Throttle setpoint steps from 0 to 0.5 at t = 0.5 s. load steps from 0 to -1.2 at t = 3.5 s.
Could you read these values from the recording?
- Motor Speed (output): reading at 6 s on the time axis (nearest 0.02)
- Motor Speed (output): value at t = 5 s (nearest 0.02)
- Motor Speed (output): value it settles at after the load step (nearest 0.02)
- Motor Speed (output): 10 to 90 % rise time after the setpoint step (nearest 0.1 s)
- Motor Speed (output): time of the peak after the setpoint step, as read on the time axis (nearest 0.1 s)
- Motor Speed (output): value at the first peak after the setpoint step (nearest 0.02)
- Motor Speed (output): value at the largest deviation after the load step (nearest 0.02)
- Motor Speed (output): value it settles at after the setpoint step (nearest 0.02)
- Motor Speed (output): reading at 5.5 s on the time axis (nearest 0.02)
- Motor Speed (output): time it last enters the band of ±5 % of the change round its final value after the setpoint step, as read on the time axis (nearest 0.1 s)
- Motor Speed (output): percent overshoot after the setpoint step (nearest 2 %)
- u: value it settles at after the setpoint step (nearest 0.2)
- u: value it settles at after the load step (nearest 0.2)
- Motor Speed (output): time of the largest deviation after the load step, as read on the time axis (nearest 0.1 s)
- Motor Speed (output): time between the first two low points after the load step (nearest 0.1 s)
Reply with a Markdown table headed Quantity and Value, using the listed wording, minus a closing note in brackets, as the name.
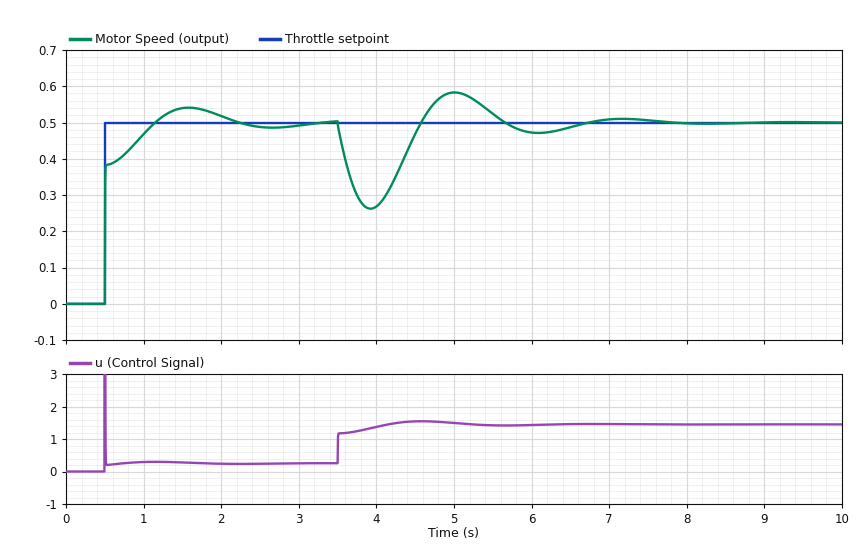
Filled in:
| Quantity | Value |
|---|---|
| Motor Speed (output): reading at 6 s on the time axis | 0.48 |
| Motor Speed (output): value at t = 5 s | 0.58 |
| Motor Speed (output): value it settles at after the load step | 0.50 |
| Motor Speed (output): 10 to 90 % rise time after the setpoint step | 0.4 s |
| Motor Speed (output): time of the peak after the setpoint step, as read on the time axis | 1.6 s |
| Motor Speed (output): value at the first peak after the setpoint step | 0.54 |
| Motor Speed (output): value at the largest deviation after the load step | 0.26 |
| Motor Speed (output): value it settles at after the setpoint step | 0.50 |
| Motor Speed (output): reading at 5.5 s on the time axis | 0.52 |
| Motor Speed (output): time it last enters the band of ±5 % of the change round its final value after the setpoint step, as read on the time axis | 1.9 s |
| Motor Speed (output): percent overshoot after the setpoint step | 8 % |
| u: value it settles at after the setpoint step | 0.2 |
| u: value it settles at after the load step | 1.4 |
| Motor Speed (output): time of the largest deviation after the load step, as read on the time axis | 3.9 s |
| Motor Speed (output): time between the first two low points after the load step | 2.2 s |
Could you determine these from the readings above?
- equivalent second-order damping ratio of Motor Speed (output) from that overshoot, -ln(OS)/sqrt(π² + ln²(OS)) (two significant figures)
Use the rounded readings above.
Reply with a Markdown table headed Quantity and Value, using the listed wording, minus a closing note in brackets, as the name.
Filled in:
| Quantity | Value |
|---|---|
| equivalent second-order damping ratio of Motor Speed (output) from that overshoot, -ln(OS)/sqrt(π² + ln²(OS)) | 0.63 |
